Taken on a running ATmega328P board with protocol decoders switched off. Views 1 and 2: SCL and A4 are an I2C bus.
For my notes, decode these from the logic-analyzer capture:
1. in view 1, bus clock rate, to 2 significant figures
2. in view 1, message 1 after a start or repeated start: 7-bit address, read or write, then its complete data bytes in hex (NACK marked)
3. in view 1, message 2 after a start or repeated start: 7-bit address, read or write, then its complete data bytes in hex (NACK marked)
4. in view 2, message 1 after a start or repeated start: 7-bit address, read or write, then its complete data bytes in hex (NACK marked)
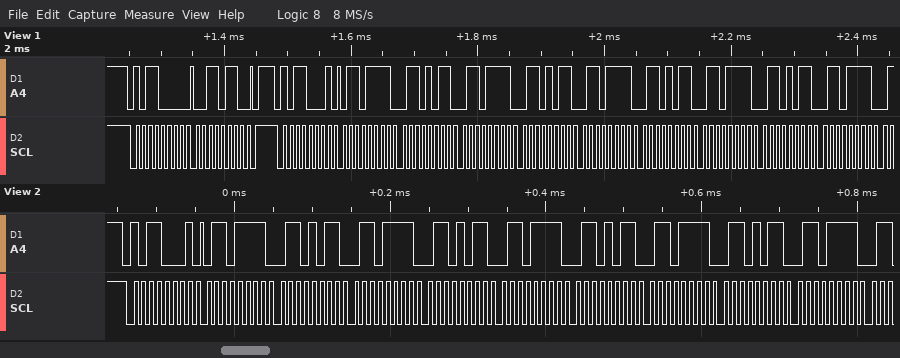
100 kHz
0x58 write: 36
0x58 read: 6F 6B 6F 6B 6F 6B 6F 6B 6F
0x58 read: 6F 6B 6F 6B 6F 6B 6F 6B 6F
